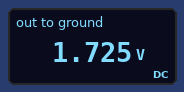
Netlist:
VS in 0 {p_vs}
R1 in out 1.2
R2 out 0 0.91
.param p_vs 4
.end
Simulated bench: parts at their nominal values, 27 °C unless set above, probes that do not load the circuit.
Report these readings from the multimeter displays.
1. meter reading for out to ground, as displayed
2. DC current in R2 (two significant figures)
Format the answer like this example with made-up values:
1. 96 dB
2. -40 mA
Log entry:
1. 1.725 V
2. 1.9 A
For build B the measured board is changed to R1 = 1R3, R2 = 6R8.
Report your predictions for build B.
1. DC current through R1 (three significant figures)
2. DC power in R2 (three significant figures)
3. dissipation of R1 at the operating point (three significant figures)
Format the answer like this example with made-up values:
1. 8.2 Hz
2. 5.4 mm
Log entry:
1. 494 mA
2. 1.66 W
3. 317 mW
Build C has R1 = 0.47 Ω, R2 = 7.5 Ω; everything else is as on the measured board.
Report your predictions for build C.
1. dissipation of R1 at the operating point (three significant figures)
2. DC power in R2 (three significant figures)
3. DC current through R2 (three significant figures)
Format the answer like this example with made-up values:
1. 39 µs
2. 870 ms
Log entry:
1. 118 mW
2. 1.89 W
3. 502 mA
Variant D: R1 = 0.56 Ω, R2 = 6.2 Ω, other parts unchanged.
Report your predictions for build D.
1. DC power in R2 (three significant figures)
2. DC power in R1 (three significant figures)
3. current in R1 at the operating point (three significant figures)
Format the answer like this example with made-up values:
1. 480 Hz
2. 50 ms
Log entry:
1. 2.17 W
2. 196 mW
3. 592 mA
